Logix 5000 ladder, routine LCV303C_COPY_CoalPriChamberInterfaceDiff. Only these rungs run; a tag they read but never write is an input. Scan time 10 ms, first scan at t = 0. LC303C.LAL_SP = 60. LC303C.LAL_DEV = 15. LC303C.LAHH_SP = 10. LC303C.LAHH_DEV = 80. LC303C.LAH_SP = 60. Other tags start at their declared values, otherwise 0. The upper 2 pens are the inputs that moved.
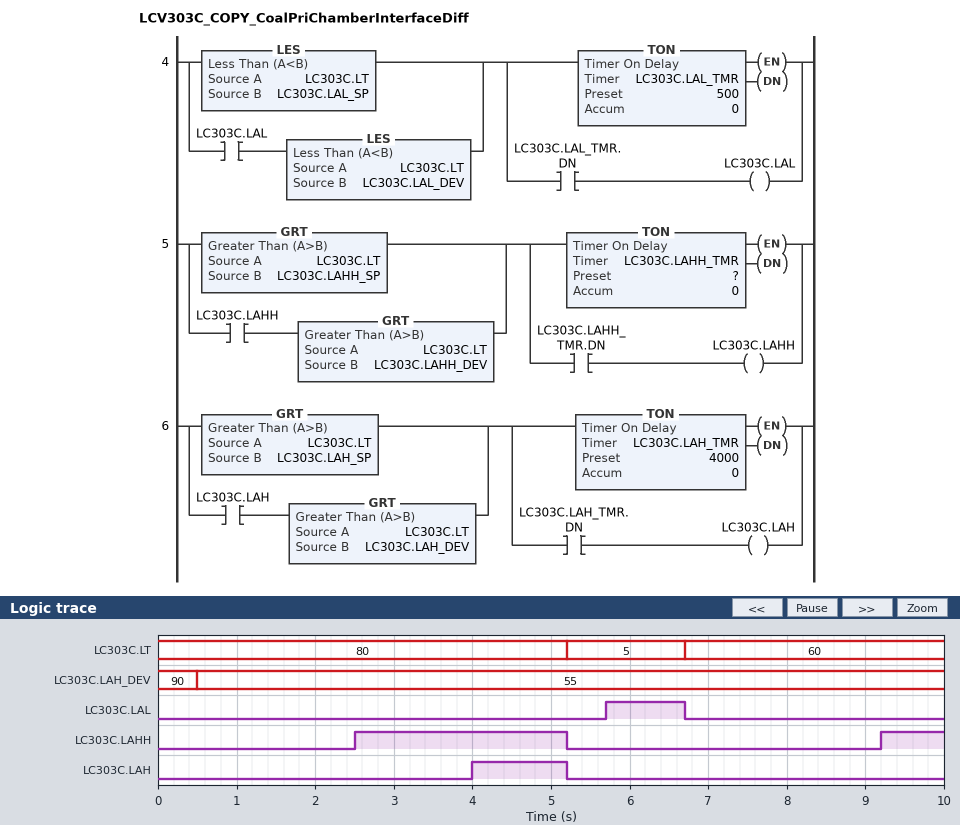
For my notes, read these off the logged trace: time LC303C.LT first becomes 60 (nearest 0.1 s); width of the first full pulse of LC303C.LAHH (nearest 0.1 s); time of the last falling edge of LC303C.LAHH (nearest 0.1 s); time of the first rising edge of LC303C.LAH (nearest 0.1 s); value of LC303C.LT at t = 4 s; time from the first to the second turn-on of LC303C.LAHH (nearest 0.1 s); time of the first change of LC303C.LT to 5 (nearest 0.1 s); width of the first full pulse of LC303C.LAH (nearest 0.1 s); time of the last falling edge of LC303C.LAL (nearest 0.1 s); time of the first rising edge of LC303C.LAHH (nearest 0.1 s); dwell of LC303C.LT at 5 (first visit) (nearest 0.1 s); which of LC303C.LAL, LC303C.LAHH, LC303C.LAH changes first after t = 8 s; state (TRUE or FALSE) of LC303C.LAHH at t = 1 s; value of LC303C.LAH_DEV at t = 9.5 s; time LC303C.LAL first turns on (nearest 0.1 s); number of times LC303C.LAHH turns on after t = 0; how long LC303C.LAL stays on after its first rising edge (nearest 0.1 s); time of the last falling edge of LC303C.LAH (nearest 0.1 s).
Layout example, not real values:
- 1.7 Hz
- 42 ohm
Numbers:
- 6.7 s
- 2.7 s
- 5.2 s
- 4.0 s
- 80
- 6.7 s
- 5.2 s
- 1.2 s
- 6.7 s
- 2.5 s
- 1.5 s
- LC303C.LAHH
- FALSE
- 55
- 5.7 s
- 2
- 1.0 s
- 5.2 s
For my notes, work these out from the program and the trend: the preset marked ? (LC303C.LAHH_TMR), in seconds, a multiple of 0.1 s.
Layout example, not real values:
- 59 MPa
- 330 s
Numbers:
- 2.5 s
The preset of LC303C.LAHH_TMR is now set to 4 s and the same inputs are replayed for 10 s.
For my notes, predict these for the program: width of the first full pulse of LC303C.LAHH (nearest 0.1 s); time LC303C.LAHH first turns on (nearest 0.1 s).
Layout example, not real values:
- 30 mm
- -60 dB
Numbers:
- 1.2 s
- 4.0 s
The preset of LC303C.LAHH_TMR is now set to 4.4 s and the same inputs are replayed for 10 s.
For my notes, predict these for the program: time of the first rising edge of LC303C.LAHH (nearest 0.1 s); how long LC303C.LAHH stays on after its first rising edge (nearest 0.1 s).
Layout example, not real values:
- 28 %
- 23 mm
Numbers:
- 4.4 s
- 0.8 s
